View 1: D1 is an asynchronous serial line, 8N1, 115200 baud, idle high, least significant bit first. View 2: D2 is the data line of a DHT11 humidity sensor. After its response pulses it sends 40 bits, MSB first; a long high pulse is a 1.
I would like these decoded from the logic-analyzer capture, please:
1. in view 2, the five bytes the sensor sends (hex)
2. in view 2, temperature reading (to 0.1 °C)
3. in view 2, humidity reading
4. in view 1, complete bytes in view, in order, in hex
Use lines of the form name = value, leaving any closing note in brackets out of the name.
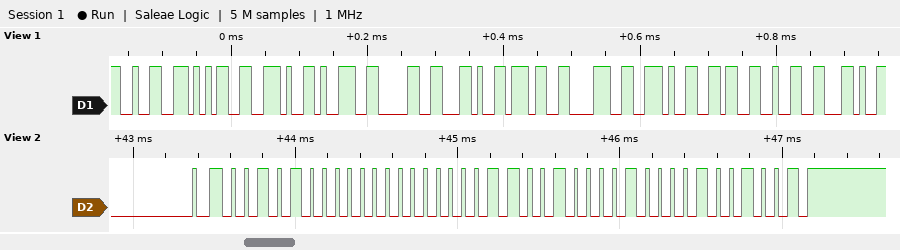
in view 2, the five bytes the sensor sends = 28 00 19 08 49
in view 2, temperature reading = 25.8 °C
in view 2, humidity reading = 40 %
in view 1, complete bytes in view, in order, in hex = 0x32 0x35 0x2E 0x39 0x30 0x2C 0x37 0x38 0x2E 0x36 0x32 0x2C
